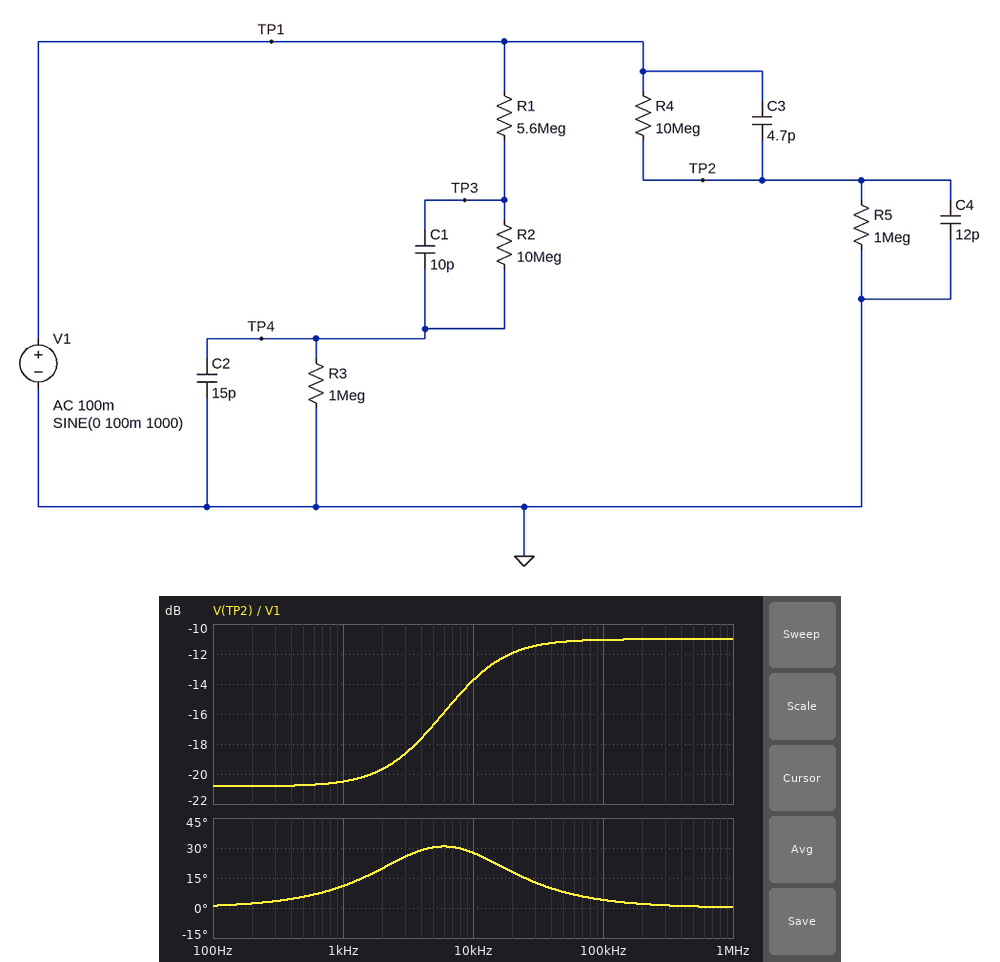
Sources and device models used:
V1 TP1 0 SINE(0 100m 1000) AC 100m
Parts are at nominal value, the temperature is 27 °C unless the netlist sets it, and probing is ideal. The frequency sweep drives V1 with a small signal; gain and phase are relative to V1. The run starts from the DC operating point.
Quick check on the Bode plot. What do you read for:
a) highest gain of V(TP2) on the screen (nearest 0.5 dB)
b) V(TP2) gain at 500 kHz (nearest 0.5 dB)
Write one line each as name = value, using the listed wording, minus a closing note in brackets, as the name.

highest gain of V(TP2) on the screen = -11.0 dB
V(TP2) gain at 500 kHz = -11.0 dB
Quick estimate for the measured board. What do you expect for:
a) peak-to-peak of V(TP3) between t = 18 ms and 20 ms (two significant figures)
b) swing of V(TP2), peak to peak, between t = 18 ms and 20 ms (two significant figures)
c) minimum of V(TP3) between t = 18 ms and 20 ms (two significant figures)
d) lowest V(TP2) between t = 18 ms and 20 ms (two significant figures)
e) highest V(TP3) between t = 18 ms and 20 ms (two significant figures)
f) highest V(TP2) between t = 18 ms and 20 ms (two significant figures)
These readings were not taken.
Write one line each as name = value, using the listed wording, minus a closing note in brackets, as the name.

peak-to-peak of V(TP3) between t = 18 ms and 20 ms = 130 mV
swing of V(TP2), peak to peak, between t = 18 ms and 20 ms = 19 mV
minimum of V(TP3) between t = 18 ms and 20 ms = -65 mV
lowest V(TP2) between t = 18 ms and 20 ms = -9.4 mV
highest V(TP3) between t = 18 ms and 20 ms = 65 mV
highest V(TP2) between t = 18 ms and 20 ms = 9.4 mV
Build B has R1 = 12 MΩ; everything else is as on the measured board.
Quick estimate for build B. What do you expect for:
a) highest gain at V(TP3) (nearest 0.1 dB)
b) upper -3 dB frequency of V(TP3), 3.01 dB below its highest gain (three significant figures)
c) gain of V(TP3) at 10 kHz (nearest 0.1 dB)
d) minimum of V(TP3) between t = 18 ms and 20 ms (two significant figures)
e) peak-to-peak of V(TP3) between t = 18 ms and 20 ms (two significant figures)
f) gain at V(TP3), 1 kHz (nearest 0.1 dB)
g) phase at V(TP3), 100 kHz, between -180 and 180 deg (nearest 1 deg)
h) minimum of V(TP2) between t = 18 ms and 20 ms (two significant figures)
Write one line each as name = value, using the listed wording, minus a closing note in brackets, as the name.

highest gain at V(TP3) = -6.4 dB
upper -3 dB frequency of V(TP3), 3.01 dB below its highest gain = 3.09 kHz
gain of V(TP3) at 10 kHz = -15.4 dB
minimum of V(TP3) between t = 18 ms and 20 ms = -45 mV
peak-to-peak of V(TP3) between t = 18 ms and 20 ms = 91 mV
gain at V(TP3), 1 kHz = -6.9 dB
phase at V(TP3), 100 kHz, between -180 and 180 deg = -86 deg
minimum of V(TP2) between t = 18 ms and 20 ms = -9.4 mV
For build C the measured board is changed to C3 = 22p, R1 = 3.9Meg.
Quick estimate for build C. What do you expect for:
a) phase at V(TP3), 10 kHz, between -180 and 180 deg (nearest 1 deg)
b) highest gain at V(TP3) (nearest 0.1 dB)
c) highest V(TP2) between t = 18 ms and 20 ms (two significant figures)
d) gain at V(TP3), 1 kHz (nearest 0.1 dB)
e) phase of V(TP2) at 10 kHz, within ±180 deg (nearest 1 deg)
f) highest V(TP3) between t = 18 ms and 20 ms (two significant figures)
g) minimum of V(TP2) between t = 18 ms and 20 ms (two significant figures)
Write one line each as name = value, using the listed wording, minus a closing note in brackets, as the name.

phase at V(TP3), 10 kHz, between -180 and 180 deg = -46 deg
highest gain at V(TP3) = -2.6 dB
highest V(TP2) between t = 18 ms and 20 ms = 15 mV
gain at V(TP3), 1 kHz = -2.8 dB
phase of V(TP2) at 10 kHz, within ±180 deg = 23 deg
highest V(TP3) between t = 18 ms and 20 ms = 73 mV
minimum of V(TP2) between t = 18 ms and 20 ms = -15 mV
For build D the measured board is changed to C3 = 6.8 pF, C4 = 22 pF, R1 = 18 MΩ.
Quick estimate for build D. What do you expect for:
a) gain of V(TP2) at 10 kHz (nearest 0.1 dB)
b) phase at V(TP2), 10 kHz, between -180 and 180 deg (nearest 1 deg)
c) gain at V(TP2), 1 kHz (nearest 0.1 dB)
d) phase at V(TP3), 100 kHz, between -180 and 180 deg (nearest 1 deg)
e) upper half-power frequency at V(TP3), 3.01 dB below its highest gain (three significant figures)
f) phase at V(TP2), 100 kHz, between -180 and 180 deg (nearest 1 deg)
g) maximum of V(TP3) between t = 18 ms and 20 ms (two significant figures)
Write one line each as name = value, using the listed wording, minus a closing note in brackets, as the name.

gain of V(TP2) at 10 kHz = -13.7 dB
phase at V(TP2), 10 kHz, between -180 and 180 deg = 18 deg
gain at V(TP2), 1 kHz = -20.2 dB
phase at V(TP3), 100 kHz, between -180 and 180 deg = -86 deg
upper half-power frequency at V(TP3), 3.01 dB below its highest gain = 2.60 kHz
phase at V(TP2), 100 kHz, between -180 and 180 deg = 2 deg
maximum of V(TP3) between t = 18 ms and 20 ms = 35 mV
